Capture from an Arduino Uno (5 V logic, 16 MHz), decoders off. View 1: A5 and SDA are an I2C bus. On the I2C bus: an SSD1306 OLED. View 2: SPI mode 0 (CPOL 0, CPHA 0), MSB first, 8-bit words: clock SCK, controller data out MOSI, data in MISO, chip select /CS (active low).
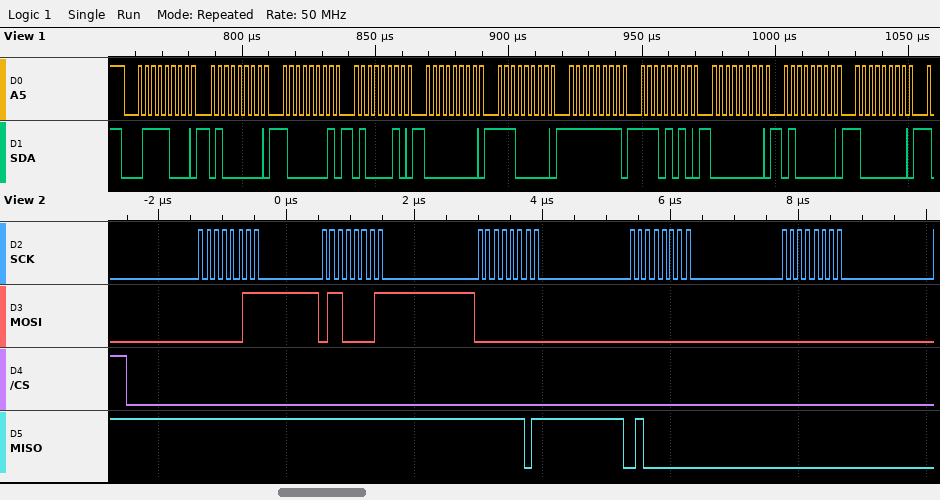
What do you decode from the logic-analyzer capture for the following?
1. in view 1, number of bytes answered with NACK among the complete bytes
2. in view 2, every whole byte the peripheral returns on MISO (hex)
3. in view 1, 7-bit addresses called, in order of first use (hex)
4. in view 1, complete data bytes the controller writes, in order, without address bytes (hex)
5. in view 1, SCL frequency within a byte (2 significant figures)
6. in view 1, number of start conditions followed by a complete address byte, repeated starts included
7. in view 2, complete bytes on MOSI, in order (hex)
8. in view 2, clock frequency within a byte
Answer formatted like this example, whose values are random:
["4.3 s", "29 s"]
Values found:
["0", "FF FF FD 40 00", "0x3C", "40 81 42 00 E0 FF EA 00 40 80", "400 kHz", "1", "03 61 00 00 00", "8 MHz"]
